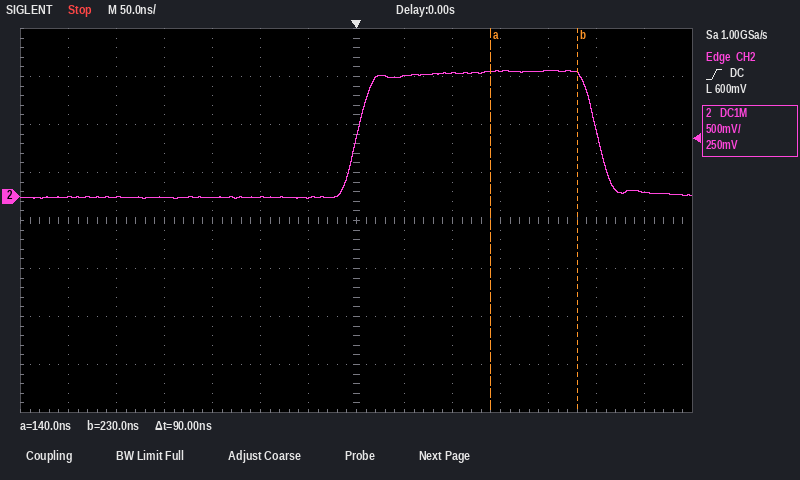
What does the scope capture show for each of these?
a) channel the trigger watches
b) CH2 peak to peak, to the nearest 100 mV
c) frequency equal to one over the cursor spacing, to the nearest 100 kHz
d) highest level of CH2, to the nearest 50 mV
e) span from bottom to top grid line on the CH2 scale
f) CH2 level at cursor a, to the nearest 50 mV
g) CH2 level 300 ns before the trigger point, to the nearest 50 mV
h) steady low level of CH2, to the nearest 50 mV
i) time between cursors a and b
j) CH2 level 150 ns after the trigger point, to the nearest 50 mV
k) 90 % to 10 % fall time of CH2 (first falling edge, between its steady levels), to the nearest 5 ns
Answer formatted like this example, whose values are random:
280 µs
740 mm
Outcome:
CH2
1.30 V
11.1 MHz
1.30 V
4 V
1.30 V
0 mV
0 mV
90 ns
1.30 V
30 ns
